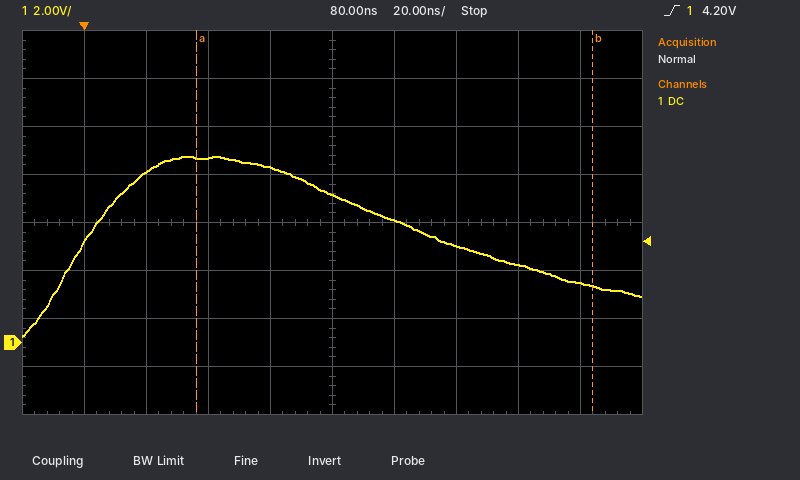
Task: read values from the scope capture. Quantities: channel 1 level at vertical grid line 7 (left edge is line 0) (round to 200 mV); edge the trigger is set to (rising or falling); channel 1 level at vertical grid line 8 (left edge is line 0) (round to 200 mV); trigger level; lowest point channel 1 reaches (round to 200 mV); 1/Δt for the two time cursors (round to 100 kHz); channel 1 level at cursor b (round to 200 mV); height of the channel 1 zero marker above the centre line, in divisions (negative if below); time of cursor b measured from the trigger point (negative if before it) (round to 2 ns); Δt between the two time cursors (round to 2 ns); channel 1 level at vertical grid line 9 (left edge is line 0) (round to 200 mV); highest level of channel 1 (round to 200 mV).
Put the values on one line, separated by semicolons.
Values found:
4.0 V; rising; 3.2 V; 4.20 V; 200 mV; 7.8 MHz; 2.4 V; -2.5 div; +164 ns; 128 ns; 2.4 V; 7.8 V
